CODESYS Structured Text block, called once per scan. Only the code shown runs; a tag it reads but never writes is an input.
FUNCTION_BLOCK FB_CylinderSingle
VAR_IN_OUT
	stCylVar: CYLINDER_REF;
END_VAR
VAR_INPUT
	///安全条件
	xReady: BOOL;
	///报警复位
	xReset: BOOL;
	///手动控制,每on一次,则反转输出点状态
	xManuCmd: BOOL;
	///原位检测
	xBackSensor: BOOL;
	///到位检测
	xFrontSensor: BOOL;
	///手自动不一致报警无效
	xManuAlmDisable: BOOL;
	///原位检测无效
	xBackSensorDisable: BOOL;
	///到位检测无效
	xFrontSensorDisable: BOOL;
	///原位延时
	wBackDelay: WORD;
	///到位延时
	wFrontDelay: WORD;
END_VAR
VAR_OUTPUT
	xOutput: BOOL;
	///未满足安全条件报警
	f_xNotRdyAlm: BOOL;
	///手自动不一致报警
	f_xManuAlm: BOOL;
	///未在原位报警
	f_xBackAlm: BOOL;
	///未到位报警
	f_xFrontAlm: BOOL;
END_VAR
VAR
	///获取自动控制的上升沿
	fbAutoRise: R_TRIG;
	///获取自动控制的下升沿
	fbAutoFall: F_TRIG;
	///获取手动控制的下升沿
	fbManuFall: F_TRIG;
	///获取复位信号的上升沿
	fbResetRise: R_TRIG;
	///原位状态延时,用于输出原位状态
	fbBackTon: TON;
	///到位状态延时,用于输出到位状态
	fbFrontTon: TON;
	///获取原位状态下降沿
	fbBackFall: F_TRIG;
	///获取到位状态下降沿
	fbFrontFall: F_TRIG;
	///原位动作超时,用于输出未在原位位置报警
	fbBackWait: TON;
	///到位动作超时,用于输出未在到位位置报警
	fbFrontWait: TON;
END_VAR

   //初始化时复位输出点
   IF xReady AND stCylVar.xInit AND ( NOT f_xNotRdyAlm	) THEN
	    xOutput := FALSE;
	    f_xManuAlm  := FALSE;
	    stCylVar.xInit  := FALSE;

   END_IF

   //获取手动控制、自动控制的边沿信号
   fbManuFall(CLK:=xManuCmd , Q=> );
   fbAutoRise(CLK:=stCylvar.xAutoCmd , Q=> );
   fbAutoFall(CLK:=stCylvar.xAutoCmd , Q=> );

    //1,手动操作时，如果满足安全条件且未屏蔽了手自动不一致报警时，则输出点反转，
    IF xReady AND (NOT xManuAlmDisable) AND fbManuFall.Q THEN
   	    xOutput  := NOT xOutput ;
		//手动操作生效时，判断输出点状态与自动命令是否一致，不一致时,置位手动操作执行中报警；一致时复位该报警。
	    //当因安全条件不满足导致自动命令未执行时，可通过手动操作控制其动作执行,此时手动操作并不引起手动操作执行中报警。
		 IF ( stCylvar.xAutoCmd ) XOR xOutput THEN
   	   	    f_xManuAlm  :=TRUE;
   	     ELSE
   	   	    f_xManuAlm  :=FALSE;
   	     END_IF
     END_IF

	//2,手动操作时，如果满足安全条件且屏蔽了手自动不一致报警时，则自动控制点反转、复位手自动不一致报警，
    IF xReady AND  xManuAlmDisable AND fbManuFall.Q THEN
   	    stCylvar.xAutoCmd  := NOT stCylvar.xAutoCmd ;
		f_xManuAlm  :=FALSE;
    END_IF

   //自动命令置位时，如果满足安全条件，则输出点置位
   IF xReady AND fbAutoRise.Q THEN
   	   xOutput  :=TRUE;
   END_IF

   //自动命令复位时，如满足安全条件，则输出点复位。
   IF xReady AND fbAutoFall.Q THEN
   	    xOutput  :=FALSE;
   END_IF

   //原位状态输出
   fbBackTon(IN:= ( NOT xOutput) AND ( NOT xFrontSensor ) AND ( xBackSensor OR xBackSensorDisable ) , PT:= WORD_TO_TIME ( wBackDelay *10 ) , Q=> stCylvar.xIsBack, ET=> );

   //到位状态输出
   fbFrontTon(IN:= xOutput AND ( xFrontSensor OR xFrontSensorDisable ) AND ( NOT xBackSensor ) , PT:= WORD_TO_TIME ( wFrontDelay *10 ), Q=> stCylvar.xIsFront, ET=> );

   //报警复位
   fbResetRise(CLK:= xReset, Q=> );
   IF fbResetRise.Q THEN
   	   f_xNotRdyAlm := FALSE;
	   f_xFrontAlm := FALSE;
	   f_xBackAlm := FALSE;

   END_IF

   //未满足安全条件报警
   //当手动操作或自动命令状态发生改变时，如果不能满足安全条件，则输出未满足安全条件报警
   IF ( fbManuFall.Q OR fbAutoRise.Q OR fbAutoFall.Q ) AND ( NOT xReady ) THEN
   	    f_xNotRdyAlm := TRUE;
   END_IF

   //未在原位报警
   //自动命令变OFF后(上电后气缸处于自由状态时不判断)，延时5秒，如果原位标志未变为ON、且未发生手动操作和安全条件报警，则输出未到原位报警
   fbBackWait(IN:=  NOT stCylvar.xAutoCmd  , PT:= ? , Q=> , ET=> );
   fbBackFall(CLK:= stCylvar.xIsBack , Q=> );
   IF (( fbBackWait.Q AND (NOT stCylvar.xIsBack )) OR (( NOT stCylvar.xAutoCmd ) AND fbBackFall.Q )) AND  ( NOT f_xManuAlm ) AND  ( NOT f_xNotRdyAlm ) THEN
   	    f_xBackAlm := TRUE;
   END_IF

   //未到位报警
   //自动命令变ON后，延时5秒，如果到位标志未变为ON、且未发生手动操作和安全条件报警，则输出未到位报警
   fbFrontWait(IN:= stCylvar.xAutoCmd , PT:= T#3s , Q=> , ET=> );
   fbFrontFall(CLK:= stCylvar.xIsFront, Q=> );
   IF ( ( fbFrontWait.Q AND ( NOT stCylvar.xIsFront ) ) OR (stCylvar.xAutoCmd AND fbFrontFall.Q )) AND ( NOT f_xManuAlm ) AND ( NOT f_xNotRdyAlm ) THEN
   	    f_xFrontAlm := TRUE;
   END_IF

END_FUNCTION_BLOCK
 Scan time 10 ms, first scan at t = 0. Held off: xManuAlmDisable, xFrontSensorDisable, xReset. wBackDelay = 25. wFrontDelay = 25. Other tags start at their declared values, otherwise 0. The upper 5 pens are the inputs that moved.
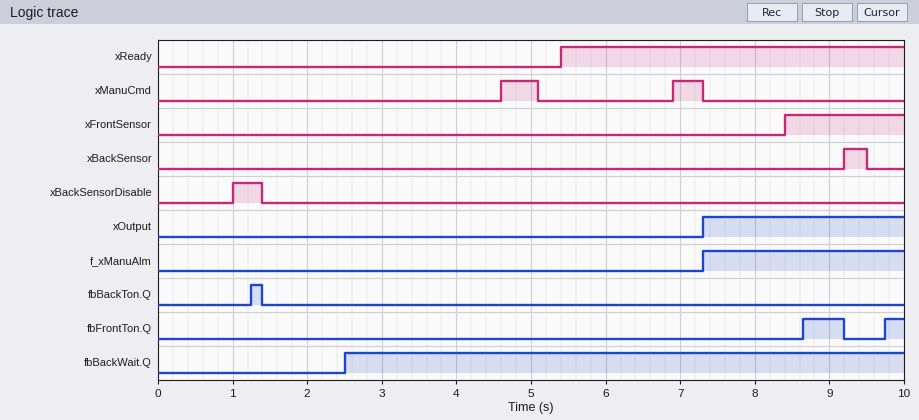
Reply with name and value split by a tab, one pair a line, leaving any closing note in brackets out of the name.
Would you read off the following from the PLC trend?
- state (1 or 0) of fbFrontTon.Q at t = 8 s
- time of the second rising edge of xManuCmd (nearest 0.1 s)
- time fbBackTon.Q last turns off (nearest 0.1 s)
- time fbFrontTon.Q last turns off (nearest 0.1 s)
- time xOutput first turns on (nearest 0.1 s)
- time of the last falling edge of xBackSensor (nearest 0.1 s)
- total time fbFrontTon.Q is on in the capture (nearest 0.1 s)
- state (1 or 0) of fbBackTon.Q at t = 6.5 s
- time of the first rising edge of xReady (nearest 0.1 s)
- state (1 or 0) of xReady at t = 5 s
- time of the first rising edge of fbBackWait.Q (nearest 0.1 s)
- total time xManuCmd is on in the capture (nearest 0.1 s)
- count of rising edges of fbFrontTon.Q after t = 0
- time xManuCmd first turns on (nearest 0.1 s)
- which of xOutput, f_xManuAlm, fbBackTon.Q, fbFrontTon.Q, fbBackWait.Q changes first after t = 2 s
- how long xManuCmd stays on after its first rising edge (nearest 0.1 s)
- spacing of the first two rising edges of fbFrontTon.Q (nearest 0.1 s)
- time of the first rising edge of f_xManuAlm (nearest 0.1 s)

state (1 or 0) of fbFrontTon.Q at t = 8 s	0
time of the second rising edge of xManuCmd	6.9 s
time fbBackTon.Q last turns off	1.4 s
time fbFrontTon.Q last turns off	9.2 s
time xOutput first turns on	7.3 s
time of the last falling edge of xBackSensor	9.5 s
total time fbFrontTon.Q is on in the capture	0.8 s
state (1 or 0) of fbBackTon.Q at t = 6.5 s	0
time of the first rising edge of xReady	5.4 s
state (1 or 0) of xReady at t = 5 s	0
time of the first rising edge of fbBackWait.Q	2.5 s
total time xManuCmd is on in the capture	0.9 s
count of rising edges of fbFrontTon.Q after t = 0	2
time xManuCmd first turns on	4.6 s
which of xOutput, f_xManuAlm, fbBackTon.Q, fbFrontTon.Q, fbBackWait.Q changes first after t = 2 s	fbBackWait.Q
how long xManuCmd stays on after its first rising edge	0.5 s
spacing of the first two rising edges of fbFrontTon.Q	1.1 s
time of the first rising edge of f_xManuAlm	7.3 s
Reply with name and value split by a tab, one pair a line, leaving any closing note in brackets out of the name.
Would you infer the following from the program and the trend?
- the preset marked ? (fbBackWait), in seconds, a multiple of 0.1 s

the preset marked ? (fbBackWait), in seconds, a multiple of 0.1 s	2.5 s
